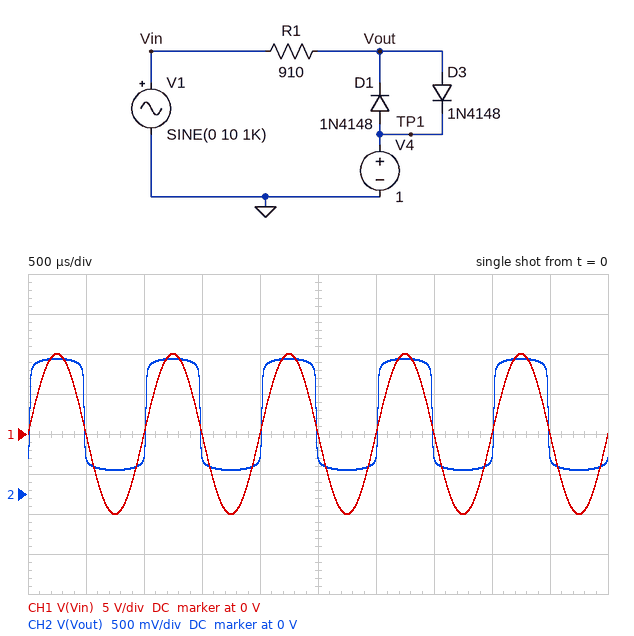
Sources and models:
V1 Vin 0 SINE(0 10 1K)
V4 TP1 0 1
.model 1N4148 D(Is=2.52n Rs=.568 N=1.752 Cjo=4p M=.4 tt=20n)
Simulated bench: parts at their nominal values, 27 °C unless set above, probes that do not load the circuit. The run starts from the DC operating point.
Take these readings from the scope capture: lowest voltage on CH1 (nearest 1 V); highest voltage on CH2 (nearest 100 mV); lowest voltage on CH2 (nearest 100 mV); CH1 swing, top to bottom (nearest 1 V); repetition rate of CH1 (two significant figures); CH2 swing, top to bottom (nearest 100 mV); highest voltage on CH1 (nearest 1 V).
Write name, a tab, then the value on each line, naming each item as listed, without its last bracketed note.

lowest voltage on CH1	-10 V
highest voltage on CH2	1.7 V
lowest voltage on CH2	300 mV
CH1 swing, top to bottom	20 V
repetition rate of CH1	1.0 kHz
CH2 swing, top to bottom	1.4 V
highest voltage on CH1	10 V
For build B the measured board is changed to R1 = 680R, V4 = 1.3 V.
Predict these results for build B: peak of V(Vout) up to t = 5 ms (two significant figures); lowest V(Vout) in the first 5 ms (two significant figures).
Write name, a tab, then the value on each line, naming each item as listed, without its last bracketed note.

peak of V(Vout) up to t = 5 ms	2.0 V
lowest V(Vout) in the first 5 ms	580 mV
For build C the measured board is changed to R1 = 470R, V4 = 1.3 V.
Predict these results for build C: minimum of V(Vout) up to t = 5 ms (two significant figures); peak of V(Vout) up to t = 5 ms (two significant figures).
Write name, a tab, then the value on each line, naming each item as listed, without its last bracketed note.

minimum of V(Vout) up to t = 5 ms	560 mV
peak of V(Vout) up to t = 5 ms	2.0 V
